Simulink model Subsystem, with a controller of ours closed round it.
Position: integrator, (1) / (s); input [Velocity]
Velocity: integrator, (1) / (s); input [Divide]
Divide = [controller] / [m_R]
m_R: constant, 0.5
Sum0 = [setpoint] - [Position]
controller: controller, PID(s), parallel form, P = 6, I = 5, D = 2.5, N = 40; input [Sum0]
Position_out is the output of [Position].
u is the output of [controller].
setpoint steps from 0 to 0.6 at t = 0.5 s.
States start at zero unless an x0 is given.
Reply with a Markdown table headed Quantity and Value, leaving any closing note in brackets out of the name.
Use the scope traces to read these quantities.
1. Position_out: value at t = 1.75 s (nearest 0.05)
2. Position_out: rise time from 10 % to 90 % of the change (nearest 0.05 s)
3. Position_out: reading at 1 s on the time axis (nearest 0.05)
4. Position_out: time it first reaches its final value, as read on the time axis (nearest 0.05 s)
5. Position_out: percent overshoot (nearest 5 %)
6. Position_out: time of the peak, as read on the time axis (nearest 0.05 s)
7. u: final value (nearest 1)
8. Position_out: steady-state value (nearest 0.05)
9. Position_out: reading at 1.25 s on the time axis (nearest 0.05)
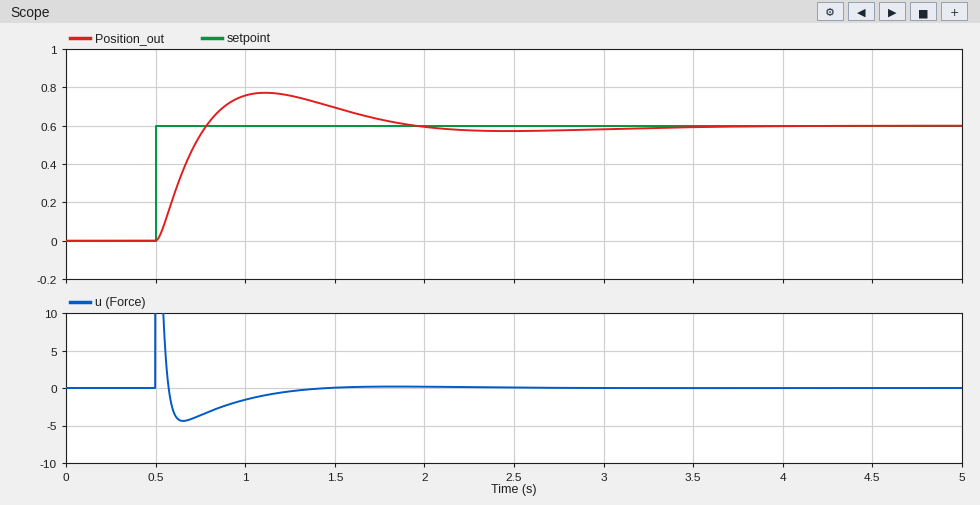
| Quantity | Value |
|---|---|
| Position_out: value at t = 1.75 s | 0.65 |
| Position_out: rise time from 10 % to 90 % of the change | 0.20 s |
| Position_out: reading at 1 s on the time axis | 0.75 |
| Position_out: time it first reaches its final value, as read on the time axis | 0.80 s |
| Position_out: percent overshoot | 30 % |
| Position_out: time of the peak, as read on the time axis | 1.10 s |
| u: final value | 0 |
| Position_out: steady-state value | 0.60 |
| Position_out: reading at 1.25 s on the time axis | 0.75 |
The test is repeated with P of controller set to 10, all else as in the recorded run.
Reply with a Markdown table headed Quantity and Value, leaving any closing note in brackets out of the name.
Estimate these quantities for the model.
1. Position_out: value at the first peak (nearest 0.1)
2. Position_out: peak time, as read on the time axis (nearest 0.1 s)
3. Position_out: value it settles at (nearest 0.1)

| Quantity | Value |
|---|---|
| Position_out: value at the first peak | 0.8 |
| Position_out: peak time, as read on the time axis | 1.0 s |
| Position_out: value it settles at | 0.6 |
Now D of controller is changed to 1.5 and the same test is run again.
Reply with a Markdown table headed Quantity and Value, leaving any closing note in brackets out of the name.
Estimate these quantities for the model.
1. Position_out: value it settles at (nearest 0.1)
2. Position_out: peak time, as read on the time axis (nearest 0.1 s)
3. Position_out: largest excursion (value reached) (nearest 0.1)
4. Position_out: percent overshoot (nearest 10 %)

| Quantity | Value |
|---|---|
| Position_out: value it settles at | 0.6 |
| Position_out: peak time, as read on the time axis | 1.2 s |
| Position_out: largest excursion (value reached) | 0.9 |
| Position_out: percent overshoot | 50 % |
